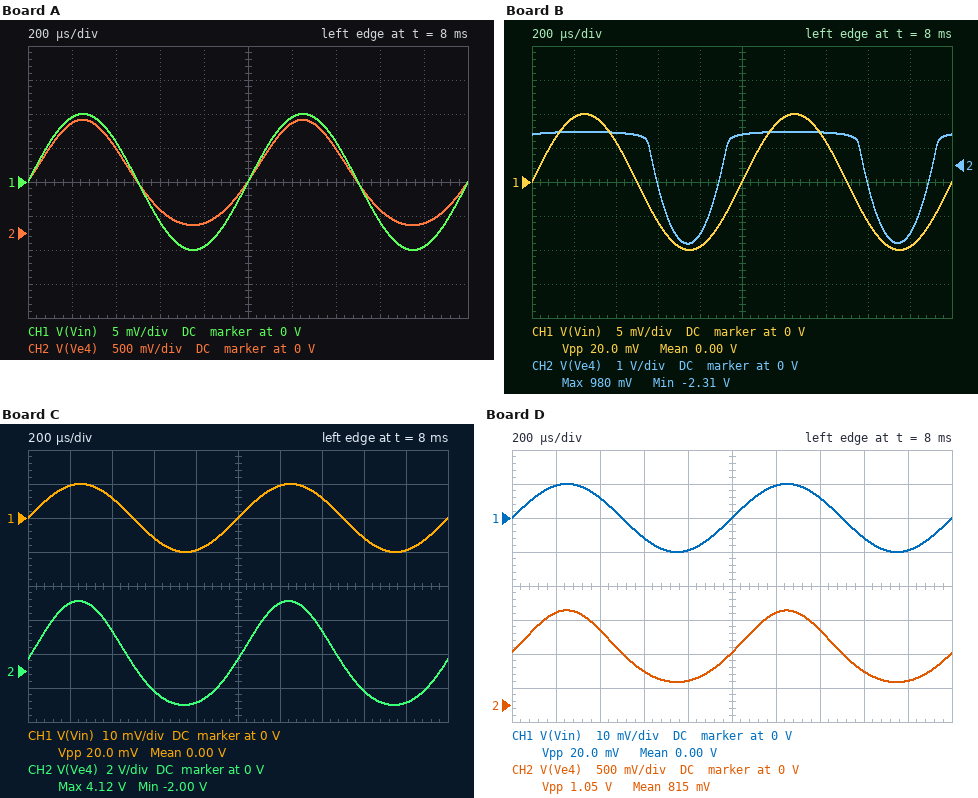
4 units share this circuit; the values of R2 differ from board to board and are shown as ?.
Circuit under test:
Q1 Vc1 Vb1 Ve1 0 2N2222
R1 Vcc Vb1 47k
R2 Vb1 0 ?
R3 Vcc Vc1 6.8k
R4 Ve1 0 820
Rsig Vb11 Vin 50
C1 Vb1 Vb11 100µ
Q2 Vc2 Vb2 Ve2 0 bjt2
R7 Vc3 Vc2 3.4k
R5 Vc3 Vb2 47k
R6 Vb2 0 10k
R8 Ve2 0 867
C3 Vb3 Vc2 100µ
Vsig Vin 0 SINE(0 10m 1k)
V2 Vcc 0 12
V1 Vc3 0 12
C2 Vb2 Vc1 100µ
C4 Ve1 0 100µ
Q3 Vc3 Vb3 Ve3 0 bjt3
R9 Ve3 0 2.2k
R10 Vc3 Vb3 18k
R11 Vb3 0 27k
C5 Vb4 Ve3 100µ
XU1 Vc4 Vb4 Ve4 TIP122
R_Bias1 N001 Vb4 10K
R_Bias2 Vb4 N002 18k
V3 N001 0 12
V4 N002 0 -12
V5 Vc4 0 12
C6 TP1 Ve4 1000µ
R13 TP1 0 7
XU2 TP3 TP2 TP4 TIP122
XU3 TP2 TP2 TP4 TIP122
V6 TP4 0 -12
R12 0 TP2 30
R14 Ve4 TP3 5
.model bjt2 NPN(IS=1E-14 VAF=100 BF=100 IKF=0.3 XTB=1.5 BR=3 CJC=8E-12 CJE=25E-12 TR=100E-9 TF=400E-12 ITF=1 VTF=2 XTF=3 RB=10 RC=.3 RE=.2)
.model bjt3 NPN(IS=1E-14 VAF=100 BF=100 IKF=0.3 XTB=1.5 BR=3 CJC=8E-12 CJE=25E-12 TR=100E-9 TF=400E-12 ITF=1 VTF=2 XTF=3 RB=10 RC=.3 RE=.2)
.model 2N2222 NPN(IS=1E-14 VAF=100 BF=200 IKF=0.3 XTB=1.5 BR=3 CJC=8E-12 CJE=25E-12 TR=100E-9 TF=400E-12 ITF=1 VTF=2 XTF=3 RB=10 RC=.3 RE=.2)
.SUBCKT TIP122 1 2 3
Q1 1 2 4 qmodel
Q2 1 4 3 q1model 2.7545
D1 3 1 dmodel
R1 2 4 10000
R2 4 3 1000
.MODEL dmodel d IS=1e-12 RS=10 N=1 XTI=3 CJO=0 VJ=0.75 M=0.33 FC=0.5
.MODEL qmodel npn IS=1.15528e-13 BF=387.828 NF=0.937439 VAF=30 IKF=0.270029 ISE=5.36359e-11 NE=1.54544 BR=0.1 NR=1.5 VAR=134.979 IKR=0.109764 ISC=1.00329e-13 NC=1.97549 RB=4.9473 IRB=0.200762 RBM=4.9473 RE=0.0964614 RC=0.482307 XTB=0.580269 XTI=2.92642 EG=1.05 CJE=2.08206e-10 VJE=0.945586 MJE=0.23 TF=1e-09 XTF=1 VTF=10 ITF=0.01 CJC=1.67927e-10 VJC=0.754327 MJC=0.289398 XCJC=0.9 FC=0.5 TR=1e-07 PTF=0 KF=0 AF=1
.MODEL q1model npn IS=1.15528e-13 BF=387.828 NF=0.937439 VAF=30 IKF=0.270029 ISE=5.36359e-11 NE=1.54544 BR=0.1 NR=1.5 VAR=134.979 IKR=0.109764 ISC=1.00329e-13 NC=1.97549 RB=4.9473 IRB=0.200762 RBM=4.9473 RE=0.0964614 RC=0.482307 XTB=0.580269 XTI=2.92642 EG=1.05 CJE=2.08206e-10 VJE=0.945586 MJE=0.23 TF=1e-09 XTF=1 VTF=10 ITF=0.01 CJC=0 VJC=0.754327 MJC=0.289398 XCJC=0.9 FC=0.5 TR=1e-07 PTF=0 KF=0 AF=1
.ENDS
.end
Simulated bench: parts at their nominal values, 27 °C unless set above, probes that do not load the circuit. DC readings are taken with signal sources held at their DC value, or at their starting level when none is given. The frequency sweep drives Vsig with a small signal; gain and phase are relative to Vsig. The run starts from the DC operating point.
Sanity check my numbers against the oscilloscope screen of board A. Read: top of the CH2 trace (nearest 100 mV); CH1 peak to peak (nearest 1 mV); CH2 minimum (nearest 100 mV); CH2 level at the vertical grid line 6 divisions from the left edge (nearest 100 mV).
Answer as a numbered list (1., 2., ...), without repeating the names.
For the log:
1. 1.7 V
2. 20 mV
3. 100 mV
4. 1.6 V
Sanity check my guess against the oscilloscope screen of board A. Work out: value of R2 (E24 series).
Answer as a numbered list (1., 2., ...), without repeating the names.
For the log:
1. 3.3 kΩ
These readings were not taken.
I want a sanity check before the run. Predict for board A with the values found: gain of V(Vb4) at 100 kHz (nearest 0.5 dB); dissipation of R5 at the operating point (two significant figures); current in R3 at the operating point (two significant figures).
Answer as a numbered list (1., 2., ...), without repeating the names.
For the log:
1. 38.0 dB
2. 2.1 mW
3. 210 µA
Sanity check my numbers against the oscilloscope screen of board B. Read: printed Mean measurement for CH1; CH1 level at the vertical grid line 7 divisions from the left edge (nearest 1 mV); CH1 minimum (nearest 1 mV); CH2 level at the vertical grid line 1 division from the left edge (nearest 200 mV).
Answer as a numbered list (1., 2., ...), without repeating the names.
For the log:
1. 0.00 V
2. 6 mV
3. -10 mV
4. 1.0 V
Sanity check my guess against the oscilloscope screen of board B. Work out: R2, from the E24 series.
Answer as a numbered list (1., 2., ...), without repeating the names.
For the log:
1. 10 kΩ
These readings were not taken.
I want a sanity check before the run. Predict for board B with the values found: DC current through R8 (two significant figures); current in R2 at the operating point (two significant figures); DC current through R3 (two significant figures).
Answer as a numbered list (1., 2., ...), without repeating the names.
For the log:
1. 1.5 mA
2. 200 µA
3. 1.6 mA
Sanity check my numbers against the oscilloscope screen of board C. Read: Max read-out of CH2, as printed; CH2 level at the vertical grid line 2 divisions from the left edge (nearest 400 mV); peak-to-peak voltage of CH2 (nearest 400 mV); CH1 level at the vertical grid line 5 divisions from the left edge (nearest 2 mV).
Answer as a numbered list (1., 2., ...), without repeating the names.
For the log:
1. 4.12 V
2. 2.4 V
3. 6.0 V
4. 0 V
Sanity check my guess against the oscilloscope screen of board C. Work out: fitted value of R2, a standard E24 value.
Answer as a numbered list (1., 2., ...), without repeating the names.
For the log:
1. 6.2 kΩ
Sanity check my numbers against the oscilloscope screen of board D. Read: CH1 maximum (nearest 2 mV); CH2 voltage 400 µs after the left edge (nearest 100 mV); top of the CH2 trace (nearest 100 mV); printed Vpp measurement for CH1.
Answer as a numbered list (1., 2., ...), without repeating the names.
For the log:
1. 10 mV
2. 1.1 V
3. 1.4 V
4. 20.0 mV
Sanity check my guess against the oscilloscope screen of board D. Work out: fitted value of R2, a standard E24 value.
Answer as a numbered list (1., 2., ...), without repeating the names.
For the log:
1. 3 kΩ
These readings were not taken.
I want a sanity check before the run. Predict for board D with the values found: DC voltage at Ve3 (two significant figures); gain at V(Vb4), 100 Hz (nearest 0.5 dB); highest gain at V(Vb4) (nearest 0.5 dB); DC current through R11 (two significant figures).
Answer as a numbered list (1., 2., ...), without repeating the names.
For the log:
1. 6.2 V
2. 34.5 dB
3. 34.5 dB
4. 260 µA
